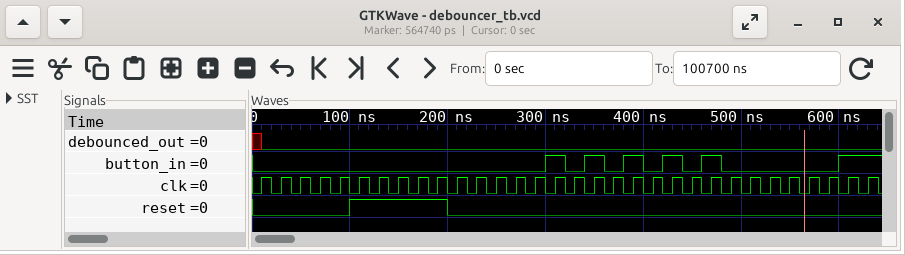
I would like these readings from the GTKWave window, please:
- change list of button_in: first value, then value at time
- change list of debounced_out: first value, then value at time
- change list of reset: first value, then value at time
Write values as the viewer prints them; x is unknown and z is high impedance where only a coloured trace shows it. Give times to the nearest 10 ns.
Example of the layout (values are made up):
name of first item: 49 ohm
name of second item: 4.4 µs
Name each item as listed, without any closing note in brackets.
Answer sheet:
change list of button_in: first value, then value at time: 0, 1 at 300 ns, 0 at 320 ns, 1 at 340 ns, 0 at 360 ns, 1 at 380 ns, 0 at 400 ns, 1 at 420 ns, 0 at 440 ns, 1 at 460 ns, 0 at 480 ns, 1 at 600 ns
change list of debounced_out: first value, then value at time: x, 0 at 10 ns
change list of reset: first value, then value at time: 0, 1 at 100 ns, 0 at 200 ns
